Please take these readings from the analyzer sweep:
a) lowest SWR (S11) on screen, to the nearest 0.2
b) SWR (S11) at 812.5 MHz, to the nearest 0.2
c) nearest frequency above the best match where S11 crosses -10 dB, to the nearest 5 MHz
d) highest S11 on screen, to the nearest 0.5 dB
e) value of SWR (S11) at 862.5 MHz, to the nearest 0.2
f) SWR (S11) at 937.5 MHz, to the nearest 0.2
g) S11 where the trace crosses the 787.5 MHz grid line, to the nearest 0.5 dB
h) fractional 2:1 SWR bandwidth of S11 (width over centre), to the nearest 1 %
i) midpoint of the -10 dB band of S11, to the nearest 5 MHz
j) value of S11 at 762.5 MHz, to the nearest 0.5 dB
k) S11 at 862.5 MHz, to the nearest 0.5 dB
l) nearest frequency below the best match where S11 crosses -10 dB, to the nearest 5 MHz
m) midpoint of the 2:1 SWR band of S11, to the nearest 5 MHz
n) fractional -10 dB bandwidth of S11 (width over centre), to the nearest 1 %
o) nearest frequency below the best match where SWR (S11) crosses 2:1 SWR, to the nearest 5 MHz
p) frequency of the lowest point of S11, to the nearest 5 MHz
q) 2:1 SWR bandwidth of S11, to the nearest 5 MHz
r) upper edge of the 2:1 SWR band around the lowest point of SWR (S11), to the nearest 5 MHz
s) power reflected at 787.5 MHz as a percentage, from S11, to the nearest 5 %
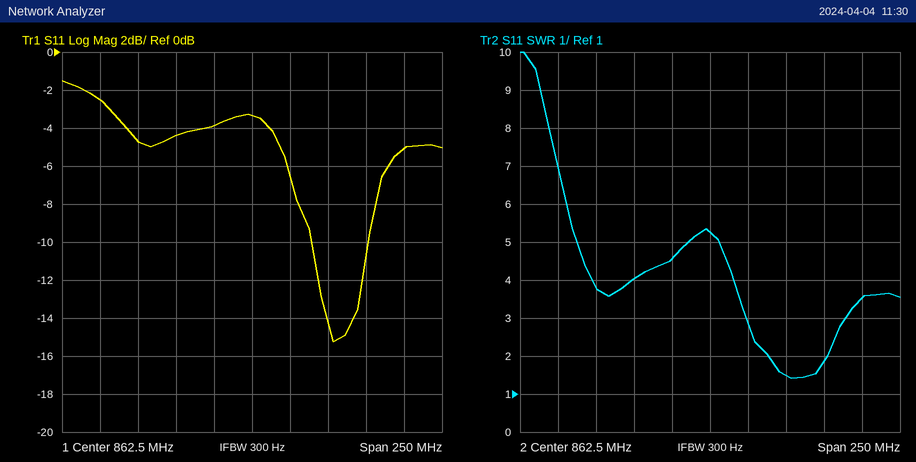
1.4
4.0
940 MHz
-1.5 dB
5.2
1.8
-4.5 dB
4 %
920 MHz
-2.5 dB
-3.5 dB
900 MHz
920 MHz
4 %
900 MHz
915 MHz
40 MHz
940 MHz
35 %
